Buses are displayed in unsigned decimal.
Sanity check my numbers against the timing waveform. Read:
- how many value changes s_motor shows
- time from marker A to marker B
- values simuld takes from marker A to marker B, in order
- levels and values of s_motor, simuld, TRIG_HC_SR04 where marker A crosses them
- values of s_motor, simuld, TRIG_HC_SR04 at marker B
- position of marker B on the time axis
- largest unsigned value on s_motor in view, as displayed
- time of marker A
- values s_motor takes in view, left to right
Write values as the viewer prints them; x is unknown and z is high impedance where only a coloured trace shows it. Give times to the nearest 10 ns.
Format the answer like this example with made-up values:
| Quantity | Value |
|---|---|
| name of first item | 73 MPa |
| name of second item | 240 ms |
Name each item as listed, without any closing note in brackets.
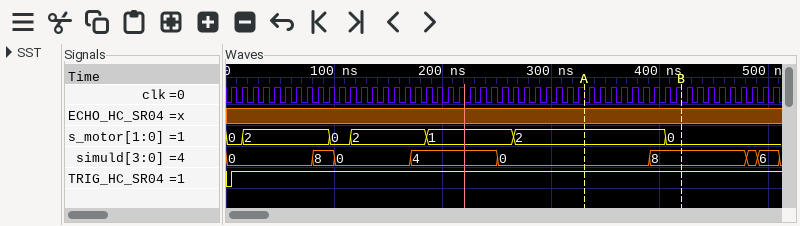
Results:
| Quantity | Value |
|---|---|
| how many value changes s_motor shows | 6 |
| time from marker A to marker B | 90 ns |
| values simuld takes from marker A to marker B, in order | 0, 8 |
| levels and values of s_motor, simuld, TRIG_HC_SR04 where marker A crosses them | s_motor=2, simuld=0, TRIG_HC_SR04=1 |
| values of s_motor, simuld, TRIG_HC_SR04 at marker B | s_motor=0, simuld=8, TRIG_HC_SR04=1 |
| position of marker B on the time axis | 420 ns |
| largest unsigned value on s_motor in view, as displayed | 2 |
| time of marker A | 330 ns |
| values s_motor takes in view, left to right | 0, 2, 0, 2, 1, 2, 0 |
